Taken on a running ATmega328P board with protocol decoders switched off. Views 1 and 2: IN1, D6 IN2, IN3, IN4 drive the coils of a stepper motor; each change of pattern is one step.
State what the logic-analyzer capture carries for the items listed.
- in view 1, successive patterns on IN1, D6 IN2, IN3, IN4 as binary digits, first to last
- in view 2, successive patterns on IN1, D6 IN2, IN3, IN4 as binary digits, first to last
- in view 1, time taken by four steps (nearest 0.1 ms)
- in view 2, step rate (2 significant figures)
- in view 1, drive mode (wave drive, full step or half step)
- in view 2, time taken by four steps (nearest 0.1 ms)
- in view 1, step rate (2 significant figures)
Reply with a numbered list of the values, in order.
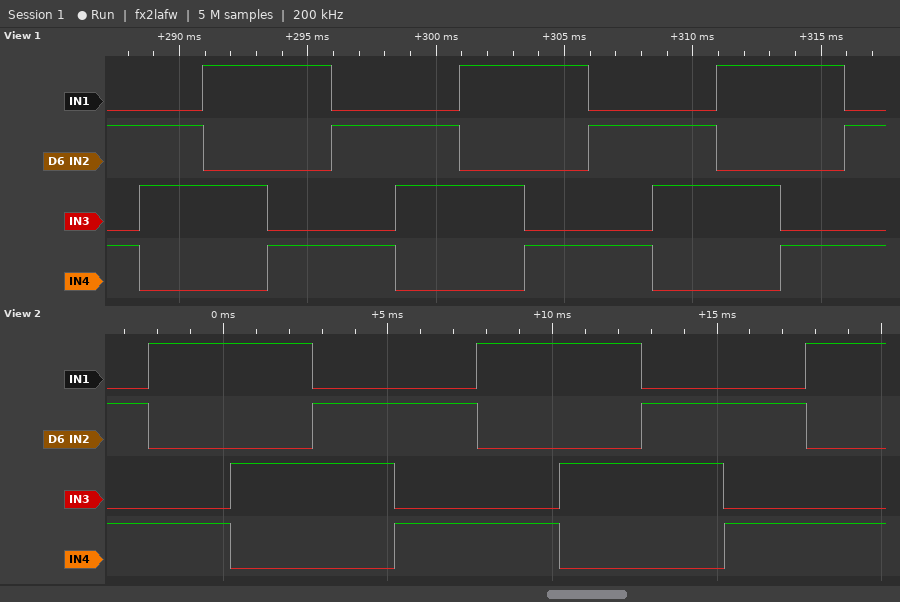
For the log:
1. 0101 0110 1010 1001 0101 0110 1010 1001 0101 0110 1010 1001 0101
2. 0101 1001 1010 0110 0101 1001 1010 0110 0101 1001
3. 10.0 ms
4. 400 steps/s
5. full step
6. 10.0 ms
7. 400 steps/s
